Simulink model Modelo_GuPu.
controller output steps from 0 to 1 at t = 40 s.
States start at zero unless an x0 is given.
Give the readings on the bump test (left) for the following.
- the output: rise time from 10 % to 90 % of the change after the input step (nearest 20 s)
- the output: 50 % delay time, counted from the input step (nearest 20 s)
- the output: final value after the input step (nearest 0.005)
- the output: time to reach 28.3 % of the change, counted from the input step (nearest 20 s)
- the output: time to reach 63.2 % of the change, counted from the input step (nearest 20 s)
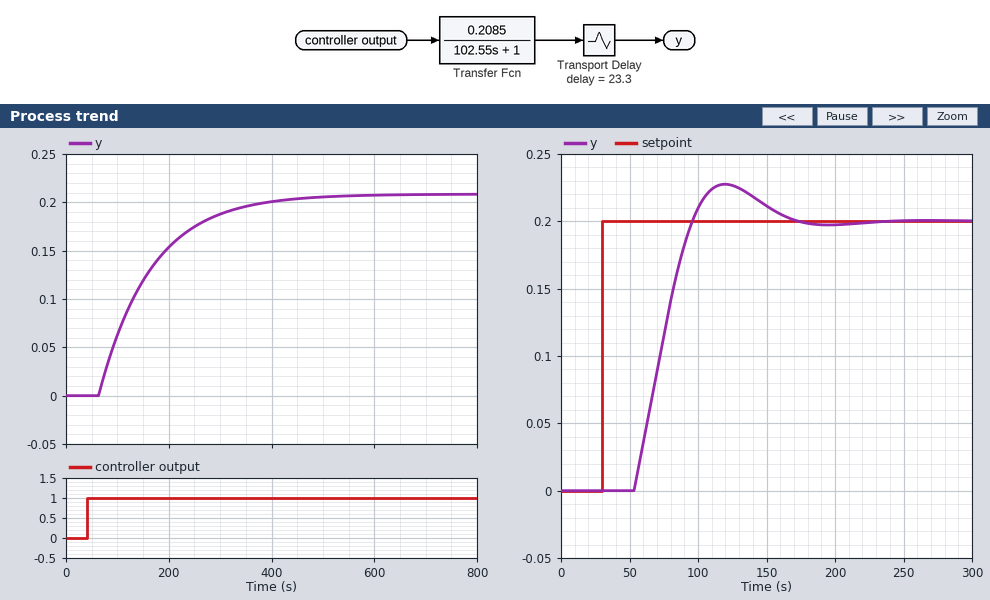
220 s
100 s
0.210
60 s
120 s
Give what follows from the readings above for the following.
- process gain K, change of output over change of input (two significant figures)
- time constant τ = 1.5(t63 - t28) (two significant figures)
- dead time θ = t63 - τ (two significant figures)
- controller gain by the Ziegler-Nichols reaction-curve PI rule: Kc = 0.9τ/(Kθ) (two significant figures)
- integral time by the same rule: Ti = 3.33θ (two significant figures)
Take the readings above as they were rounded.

0.21
90 s
30 s
13
100 s
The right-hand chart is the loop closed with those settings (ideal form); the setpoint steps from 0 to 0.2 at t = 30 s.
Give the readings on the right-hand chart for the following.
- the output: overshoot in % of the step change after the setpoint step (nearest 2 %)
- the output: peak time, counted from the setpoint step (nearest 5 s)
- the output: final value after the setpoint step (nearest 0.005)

14 %
90 s
0.200
